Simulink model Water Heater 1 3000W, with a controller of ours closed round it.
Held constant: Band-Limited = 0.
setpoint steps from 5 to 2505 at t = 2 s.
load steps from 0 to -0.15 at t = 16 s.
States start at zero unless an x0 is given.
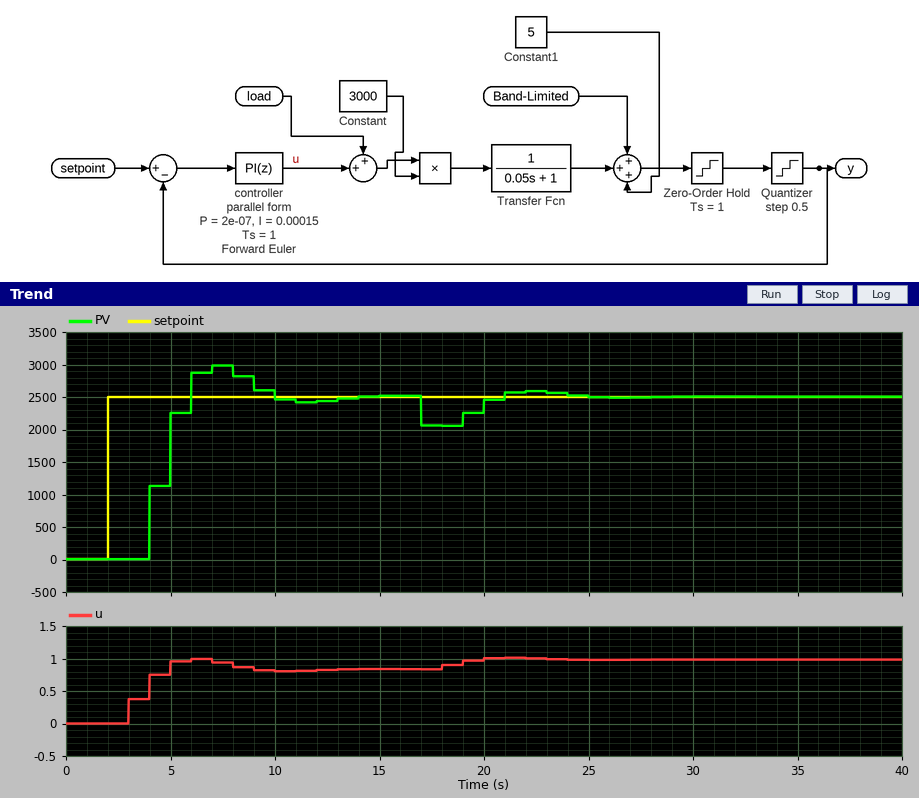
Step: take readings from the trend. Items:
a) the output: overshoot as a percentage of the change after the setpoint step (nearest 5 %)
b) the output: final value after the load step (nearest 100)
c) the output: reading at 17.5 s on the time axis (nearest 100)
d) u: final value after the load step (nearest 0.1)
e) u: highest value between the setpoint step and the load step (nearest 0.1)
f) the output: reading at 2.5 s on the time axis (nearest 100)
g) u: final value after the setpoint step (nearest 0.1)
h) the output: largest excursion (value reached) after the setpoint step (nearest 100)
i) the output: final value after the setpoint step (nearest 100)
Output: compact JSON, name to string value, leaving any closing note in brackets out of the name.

{"the output: overshoot as a percentage of the change after the setpoint step": "20 %", "the output: final value after the load step": "2500", "the output: reading at 17.5 s on the time axis": "2100", "u: final value after the load step": "1.0", "u: highest value between the setpoint step and the load step": "1.0", "the output: reading at 2.5 s on the time axis": "0", "u: final value after the setpoint step": "0.8", "the output: largest excursion (value reached) after the setpoint step": "3000", "the output: final value after the setpoint step": "2500"}
